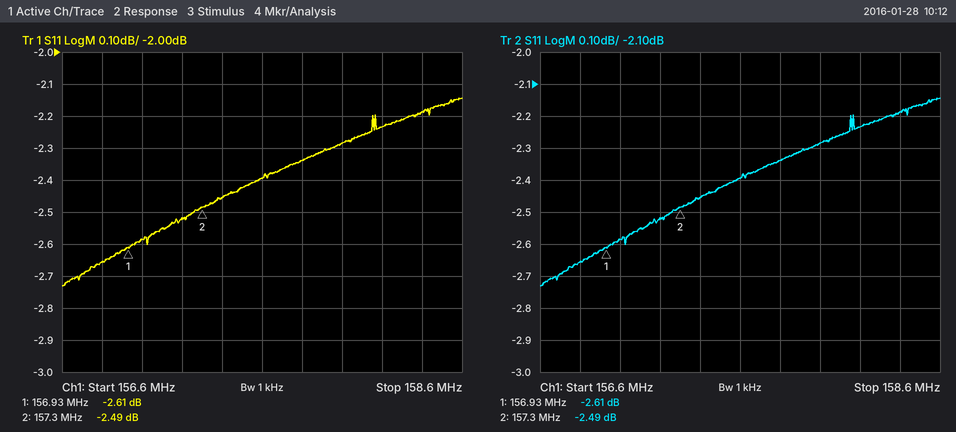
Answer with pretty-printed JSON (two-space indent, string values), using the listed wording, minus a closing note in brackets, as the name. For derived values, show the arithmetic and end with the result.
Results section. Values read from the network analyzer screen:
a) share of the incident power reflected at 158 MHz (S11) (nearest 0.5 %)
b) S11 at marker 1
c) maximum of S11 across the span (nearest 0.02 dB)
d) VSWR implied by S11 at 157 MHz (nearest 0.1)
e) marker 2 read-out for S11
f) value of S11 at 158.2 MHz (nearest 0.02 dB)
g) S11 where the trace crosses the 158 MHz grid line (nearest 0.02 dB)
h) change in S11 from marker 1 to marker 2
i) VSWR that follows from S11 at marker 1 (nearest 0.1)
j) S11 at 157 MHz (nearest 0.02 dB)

{
  "share of the incident power reflected at 158 MHz (S11)": "10^(-2.28/10) ≈ 59.2 %, so 59.0 % to the nearest 0.5 %",
  "S11 at marker 1": "-2.61 dB",
  "maximum of S11 across the span": "-2.14 dB",
  "VSWR implied by S11 at 157 MHz": "|Γ| = 10^(-2.58/20) = 0.7430; VSWR = (1 + 0.7430)/(1 − 0.7430) ≈ 6.8",
  "marker 2 read-out for S11": "-2.49 dB",
  "value of S11 at 158.2 MHz": "-2.24 dB",
  "S11 where the trace crosses the 158 MHz grid line": "-2.28 dB",
  "change in S11 from marker 1 to marker 2": "-2.49 − (-2.61) = 0.12 dB",
  "VSWR that follows from S11 at marker 1": "(1 + 0.7405)/(1 − 0.7405) ≈ 6.7",
  "S11 at 157 MHz": "-2.58 dB"
}
